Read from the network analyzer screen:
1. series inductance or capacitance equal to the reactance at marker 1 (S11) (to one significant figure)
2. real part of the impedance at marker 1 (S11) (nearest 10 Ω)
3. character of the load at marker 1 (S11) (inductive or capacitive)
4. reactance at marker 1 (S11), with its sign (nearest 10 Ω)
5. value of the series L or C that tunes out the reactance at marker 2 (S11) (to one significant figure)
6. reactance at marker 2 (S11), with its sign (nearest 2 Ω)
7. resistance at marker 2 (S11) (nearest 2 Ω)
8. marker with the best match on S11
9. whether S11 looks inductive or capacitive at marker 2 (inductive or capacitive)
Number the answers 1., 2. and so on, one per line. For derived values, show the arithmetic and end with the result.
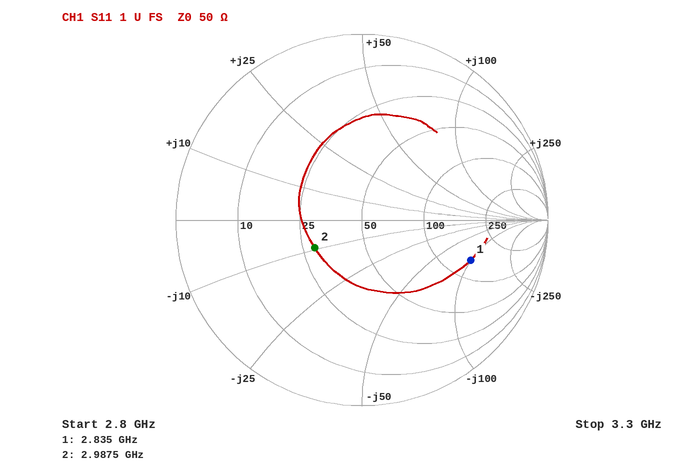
1. C = 1/(2π × 2.835 GHz × 100 Ω) ≈ 561 fF, so 600 fF to one significant figure
2. 140 Ω
3. capacitive
4. -100 Ω
5. L = 10 Ω/(2π × 2.9875 GHz) ≈ 533 pH, so 500 pH to one significant figure
6. -10 Ω
7. 28 Ω
8. marker 2
9. capacitive
